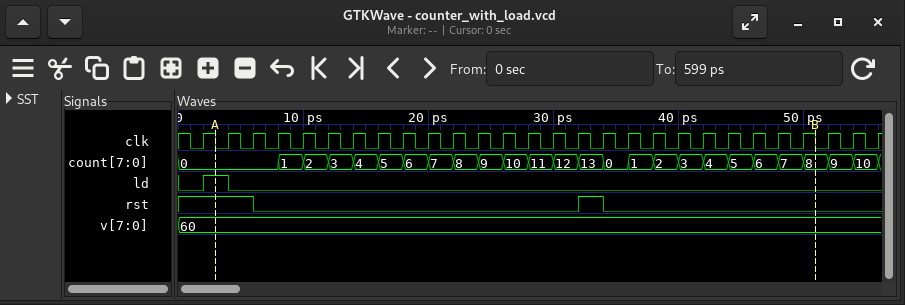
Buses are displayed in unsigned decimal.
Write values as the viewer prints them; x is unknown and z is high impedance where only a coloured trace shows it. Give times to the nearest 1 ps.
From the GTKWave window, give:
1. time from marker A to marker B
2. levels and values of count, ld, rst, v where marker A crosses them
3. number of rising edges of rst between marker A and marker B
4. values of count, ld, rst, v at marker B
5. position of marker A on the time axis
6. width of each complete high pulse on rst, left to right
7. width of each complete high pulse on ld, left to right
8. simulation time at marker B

48 ps
count=0, ld=1, rst=1, v=60
1
count=8, ld=0, rst=0, v=60
3 ps
2 ps
2 ps
51 ps
